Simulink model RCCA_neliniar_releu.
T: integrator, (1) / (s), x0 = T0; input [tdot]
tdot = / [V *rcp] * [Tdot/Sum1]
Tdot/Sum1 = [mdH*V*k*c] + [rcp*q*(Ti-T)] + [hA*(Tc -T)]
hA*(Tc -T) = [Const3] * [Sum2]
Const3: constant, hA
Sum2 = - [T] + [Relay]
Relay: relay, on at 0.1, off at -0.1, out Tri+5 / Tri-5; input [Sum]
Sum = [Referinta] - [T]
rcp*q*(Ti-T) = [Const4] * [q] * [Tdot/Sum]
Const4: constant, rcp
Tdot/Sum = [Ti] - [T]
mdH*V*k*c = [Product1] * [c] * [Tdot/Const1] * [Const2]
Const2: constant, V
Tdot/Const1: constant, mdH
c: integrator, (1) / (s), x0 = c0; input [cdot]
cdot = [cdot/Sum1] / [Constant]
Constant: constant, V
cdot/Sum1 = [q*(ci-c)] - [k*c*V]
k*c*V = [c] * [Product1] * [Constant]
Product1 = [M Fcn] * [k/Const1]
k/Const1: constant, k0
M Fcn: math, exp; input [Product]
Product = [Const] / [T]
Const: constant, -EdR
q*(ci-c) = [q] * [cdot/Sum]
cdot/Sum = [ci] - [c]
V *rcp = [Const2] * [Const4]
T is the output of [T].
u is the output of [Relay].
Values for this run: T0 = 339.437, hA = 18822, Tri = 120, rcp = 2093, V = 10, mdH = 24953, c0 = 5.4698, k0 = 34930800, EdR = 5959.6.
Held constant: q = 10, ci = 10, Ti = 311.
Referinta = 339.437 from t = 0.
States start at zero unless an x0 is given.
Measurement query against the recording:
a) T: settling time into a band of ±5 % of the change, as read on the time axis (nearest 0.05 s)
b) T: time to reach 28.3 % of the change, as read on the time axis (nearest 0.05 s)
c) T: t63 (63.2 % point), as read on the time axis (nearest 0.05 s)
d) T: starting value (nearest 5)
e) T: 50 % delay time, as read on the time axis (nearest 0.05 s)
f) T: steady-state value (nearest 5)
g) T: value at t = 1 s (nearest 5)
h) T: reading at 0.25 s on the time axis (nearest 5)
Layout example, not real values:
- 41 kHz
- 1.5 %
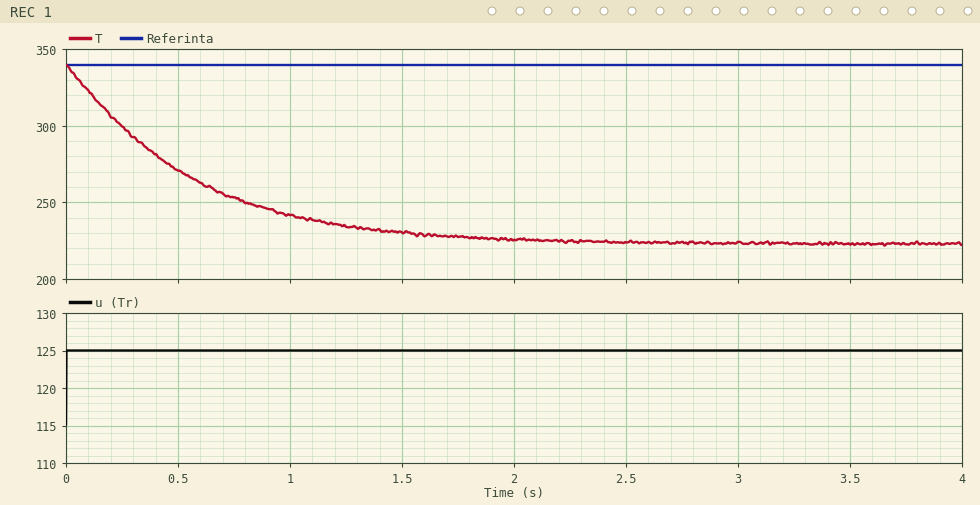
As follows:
- 1.60 s
- 0.20 s
- 0.55 s
- 340
- 0.40 s
- 225
- 240
- 300
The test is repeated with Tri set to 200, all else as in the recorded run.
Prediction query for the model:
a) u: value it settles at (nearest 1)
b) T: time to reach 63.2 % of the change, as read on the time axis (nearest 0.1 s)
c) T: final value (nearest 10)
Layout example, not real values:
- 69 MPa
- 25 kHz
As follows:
- 205
- 0.6 s
- 260
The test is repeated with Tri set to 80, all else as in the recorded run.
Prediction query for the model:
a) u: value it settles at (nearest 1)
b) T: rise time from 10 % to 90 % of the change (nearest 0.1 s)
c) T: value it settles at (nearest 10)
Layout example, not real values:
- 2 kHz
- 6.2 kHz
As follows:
- 85
- 1.2 s
- 200
